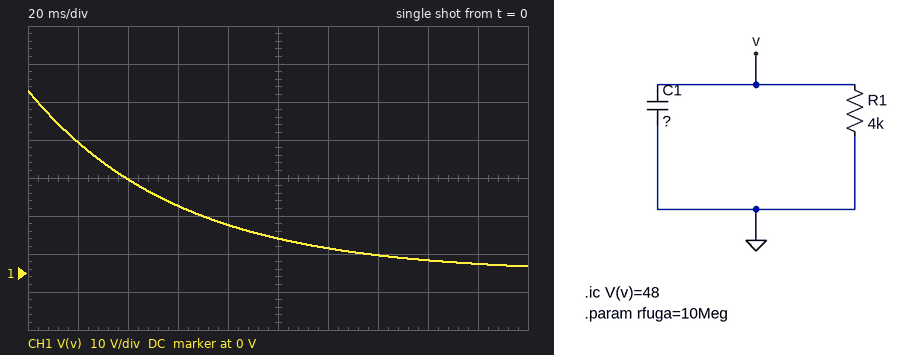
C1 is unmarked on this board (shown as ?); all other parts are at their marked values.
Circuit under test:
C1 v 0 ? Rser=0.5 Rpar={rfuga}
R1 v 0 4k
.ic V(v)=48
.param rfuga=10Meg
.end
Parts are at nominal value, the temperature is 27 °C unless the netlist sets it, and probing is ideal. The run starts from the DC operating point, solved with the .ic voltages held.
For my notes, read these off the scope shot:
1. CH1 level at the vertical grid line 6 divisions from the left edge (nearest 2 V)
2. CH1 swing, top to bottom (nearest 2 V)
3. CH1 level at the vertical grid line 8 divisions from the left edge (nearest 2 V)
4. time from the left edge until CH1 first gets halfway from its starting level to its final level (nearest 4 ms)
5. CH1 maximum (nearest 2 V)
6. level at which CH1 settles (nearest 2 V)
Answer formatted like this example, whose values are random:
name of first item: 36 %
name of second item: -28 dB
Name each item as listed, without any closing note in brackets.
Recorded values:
CH1 level at the vertical grid line 6 divisions from the left edge: 6 V
CH1 swing, top to bottom: 46 V
CH1 level at the vertical grid line 8 divisions from the left edge: 4 V
time from the left edge until CH1 first gets halfway from its starting level to its final level: 40 ms
CH1 maximum: 48 V
level at which CH1 settles: 2 V
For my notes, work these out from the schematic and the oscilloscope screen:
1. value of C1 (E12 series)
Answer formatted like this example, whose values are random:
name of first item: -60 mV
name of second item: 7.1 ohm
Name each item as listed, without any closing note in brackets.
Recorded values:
value of C1: 15 µF
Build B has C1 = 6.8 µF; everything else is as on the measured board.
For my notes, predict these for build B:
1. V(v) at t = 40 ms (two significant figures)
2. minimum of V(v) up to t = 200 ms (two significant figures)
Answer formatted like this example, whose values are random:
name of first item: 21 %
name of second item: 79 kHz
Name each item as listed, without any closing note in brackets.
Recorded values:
V(v) at t = 40 ms: 11 V
minimum of V(v) up to t = 200 ms: 31 mV
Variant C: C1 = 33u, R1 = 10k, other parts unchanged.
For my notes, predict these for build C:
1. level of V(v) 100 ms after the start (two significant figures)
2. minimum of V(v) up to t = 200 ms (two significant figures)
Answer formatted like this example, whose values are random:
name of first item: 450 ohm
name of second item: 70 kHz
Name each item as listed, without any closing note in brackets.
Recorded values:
level of V(v) 100 ms after the start: 35 V
minimum of V(v) up to t = 200 ms: 26 V
